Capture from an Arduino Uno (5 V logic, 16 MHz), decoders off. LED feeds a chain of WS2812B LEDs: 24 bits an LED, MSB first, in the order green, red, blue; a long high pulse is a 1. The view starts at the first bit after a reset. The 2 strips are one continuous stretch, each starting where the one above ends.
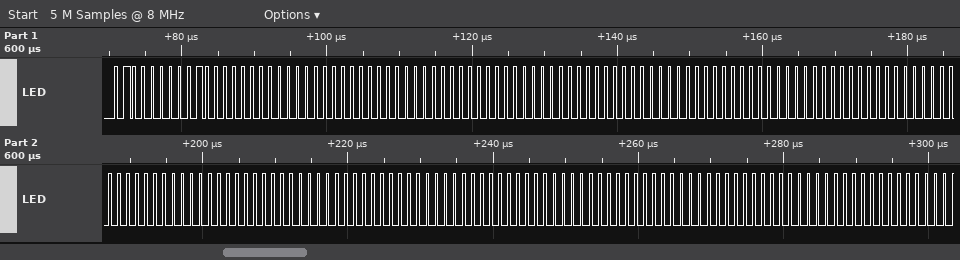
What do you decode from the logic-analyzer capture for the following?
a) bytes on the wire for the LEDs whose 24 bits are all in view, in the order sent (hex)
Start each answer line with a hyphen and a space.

- 40 40 00 00 00 00 00 00 00 00 00 00 00 00 00 00 00 00 00 00 00
